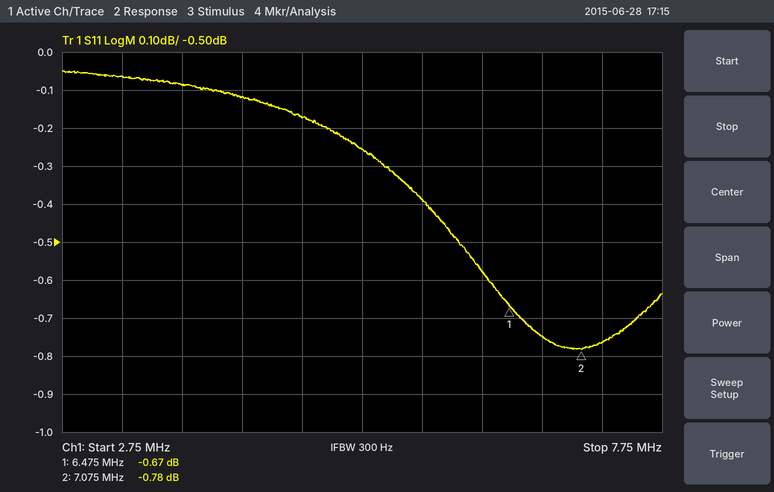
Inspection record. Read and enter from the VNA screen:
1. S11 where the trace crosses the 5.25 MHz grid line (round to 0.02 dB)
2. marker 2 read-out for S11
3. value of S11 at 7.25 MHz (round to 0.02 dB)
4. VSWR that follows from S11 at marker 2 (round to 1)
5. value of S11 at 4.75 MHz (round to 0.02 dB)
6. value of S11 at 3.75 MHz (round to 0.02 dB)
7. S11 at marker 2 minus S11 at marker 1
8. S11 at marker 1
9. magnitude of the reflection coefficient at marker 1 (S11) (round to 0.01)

-0.26 dB
-0.78 dB
-0.76 dB
22
-0.18 dB
-0.08 dB
-0.11 dB
-0.67 dB
0.93
